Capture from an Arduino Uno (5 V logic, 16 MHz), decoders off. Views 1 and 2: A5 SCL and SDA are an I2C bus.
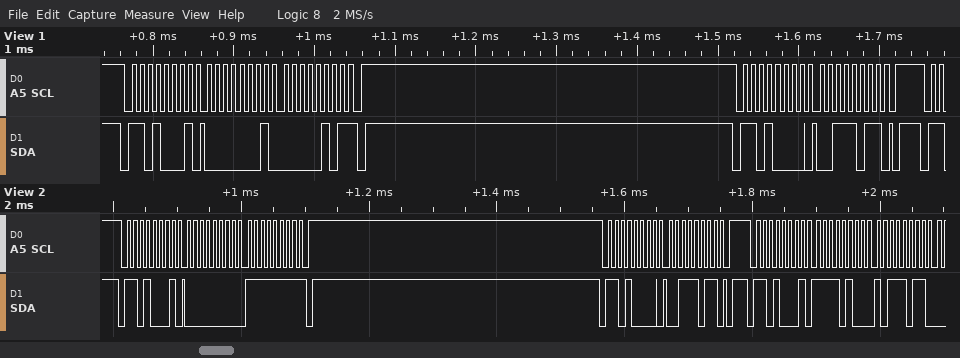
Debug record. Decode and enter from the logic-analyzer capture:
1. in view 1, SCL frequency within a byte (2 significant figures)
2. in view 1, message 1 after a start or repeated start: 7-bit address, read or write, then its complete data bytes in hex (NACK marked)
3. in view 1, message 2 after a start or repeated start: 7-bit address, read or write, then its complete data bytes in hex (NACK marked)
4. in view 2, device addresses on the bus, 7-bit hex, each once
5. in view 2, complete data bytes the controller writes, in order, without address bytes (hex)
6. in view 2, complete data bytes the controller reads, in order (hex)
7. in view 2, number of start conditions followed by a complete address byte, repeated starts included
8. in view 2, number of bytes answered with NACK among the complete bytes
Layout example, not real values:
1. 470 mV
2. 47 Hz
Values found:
1. 100 kHz
2. 0x68 read: 01 05 NACK
3. 0x68 write: 3B
4. 0x68
5. 3B
6. 00 FF F4 BB
7. 3
8. 1
